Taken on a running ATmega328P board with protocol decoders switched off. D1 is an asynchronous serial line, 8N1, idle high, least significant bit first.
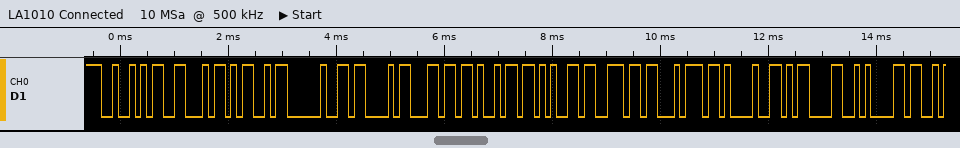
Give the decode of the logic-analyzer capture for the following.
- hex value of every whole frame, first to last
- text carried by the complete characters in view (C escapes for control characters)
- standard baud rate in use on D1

0x52 0x46 0x4D 0x20 0x43 0x6C 0x69 0x65 0x6E 0x74 0x21 0x0D 0x0A
"RFM Client!\r\n"
9600 baud
